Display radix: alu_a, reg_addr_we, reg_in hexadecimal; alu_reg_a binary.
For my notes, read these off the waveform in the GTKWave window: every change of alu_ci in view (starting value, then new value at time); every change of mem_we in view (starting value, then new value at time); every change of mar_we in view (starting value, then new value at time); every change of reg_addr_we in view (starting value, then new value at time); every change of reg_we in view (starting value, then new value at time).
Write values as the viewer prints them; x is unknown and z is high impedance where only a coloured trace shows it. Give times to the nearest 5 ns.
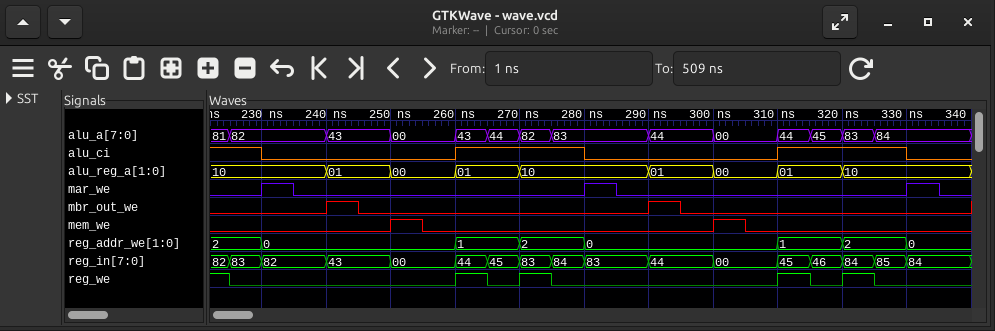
1, 0 at 230 ns, 1 at 260 ns, 0 at 280 ns, 1 at 310 ns, 0 at 330 ns
0, 1 at 250 ns, 0 at 255 ns, 1 at 300 ns, 0 at 305 ns
0, 1 at 230 ns, 0 at 235 ns, 1 at 280 ns, 0 at 285 ns, 1 at 330 ns, 0 at 335 ns
2, 0 at 230 ns, 1 at 260 ns, 2 at 270 ns, 0 at 280 ns, 1 at 310 ns, 2 at 320 ns, 0 at 330 ns
1, 0 at 225 ns, 1 at 260 ns, 0 at 265 ns, 1 at 270 ns, 0 at 275 ns, 1 at 310 ns, 0 at 315 ns, 1 at 320 ns, 0 at 325 ns
